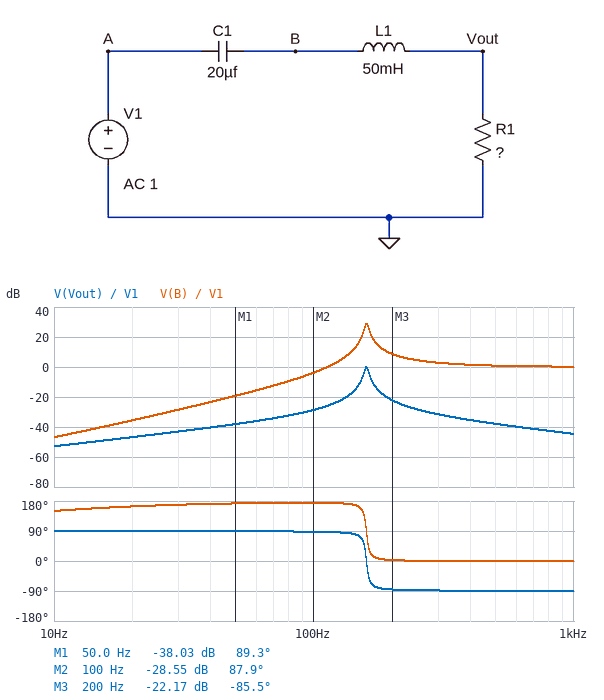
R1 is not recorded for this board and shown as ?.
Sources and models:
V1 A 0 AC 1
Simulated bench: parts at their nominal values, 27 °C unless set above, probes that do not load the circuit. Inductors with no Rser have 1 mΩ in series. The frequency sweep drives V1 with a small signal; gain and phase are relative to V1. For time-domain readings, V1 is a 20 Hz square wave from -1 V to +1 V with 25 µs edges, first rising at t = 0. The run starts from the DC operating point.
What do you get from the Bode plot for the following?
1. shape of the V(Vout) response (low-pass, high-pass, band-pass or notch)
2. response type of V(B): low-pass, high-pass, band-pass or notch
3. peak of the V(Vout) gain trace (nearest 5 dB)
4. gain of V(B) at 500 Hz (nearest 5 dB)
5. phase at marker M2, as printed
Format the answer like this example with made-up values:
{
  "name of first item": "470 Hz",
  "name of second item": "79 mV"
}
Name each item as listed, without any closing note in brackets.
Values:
{
  "shape of the V(Vout) response": "band-pass",
  "response type of V(B): low-pass, high-pass, band-pass or notch": "high-pass",
  "peak of the V(Vout) gain trace": "0 dB",
  "gain of V(B) at 500 Hz": "0 dB",
  "phase at marker M2, as printed": "87.9 deg"
}
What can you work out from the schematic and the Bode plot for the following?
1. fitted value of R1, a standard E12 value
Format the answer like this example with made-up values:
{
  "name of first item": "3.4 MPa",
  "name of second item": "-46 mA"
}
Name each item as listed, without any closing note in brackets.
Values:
{
  "fitted value of R1, a standard E12 value": "1.8 Ω"
}
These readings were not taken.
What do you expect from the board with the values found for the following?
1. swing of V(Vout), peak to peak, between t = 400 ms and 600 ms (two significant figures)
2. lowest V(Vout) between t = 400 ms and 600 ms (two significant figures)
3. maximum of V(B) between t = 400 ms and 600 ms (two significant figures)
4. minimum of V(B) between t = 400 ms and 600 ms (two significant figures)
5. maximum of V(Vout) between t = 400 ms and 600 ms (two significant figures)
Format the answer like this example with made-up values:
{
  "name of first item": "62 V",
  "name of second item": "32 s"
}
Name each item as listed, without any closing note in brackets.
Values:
{
  "swing of V(Vout), peak to peak, between t = 400 ms and 600 ms": "86 mV",
  "lowest V(Vout) between t = 400 ms and 600 ms": "-43 mV",
  "maximum of V(B) between t = 400 ms and 600 ms": "1.2 V",
  "minimum of V(B) between t = 400 ms and 600 ms": "-1.2 V",
  "maximum of V(Vout) between t = 400 ms and 600 ms": "43 mV"
}
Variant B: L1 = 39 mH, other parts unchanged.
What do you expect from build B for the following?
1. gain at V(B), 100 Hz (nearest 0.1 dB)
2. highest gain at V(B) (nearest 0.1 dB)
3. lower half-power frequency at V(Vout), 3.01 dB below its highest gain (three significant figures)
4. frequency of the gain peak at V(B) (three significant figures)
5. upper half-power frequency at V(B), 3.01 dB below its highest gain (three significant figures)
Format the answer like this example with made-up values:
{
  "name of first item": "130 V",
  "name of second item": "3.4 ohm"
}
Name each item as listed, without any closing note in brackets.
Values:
{
  "gain at V(B), 100 Hz": "-7.0 dB",
  "highest gain at V(B)": "27.8 dB",
  "lower half-power frequency at V(Vout), 3.01 dB below its highest gain": "177 Hz",
  "frequency of the gain peak at V(B)": "180 Hz",
  "upper half-power frequency at V(B), 3.01 dB below its highest gain": "184 Hz"
}
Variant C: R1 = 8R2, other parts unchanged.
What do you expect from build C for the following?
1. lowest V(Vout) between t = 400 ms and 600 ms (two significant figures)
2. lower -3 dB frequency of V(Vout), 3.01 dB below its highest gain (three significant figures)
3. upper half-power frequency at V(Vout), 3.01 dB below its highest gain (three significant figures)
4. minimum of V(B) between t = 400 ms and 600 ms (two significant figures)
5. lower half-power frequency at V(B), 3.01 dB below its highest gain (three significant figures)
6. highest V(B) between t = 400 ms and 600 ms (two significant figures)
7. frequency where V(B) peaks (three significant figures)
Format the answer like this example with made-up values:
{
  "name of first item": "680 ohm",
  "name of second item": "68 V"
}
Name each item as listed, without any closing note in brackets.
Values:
{
  "lowest V(Vout) between t = 400 ms and 600 ms": "-260 mV",
  "lower -3 dB frequency of V(Vout), 3.01 dB below its highest gain": "147 Hz",
  "upper half-power frequency at V(Vout), 3.01 dB below its highest gain": "173 Hz",
  "minimum of V(B) between t = 400 ms and 600 ms": "-1.8 V",
  "lower half-power frequency at V(B), 3.01 dB below its highest gain": "148 Hz",
  "highest V(B) between t = 400 ms and 600 ms": "1.8 V",
  "frequency where V(B) peaks": "160 Hz"
}
